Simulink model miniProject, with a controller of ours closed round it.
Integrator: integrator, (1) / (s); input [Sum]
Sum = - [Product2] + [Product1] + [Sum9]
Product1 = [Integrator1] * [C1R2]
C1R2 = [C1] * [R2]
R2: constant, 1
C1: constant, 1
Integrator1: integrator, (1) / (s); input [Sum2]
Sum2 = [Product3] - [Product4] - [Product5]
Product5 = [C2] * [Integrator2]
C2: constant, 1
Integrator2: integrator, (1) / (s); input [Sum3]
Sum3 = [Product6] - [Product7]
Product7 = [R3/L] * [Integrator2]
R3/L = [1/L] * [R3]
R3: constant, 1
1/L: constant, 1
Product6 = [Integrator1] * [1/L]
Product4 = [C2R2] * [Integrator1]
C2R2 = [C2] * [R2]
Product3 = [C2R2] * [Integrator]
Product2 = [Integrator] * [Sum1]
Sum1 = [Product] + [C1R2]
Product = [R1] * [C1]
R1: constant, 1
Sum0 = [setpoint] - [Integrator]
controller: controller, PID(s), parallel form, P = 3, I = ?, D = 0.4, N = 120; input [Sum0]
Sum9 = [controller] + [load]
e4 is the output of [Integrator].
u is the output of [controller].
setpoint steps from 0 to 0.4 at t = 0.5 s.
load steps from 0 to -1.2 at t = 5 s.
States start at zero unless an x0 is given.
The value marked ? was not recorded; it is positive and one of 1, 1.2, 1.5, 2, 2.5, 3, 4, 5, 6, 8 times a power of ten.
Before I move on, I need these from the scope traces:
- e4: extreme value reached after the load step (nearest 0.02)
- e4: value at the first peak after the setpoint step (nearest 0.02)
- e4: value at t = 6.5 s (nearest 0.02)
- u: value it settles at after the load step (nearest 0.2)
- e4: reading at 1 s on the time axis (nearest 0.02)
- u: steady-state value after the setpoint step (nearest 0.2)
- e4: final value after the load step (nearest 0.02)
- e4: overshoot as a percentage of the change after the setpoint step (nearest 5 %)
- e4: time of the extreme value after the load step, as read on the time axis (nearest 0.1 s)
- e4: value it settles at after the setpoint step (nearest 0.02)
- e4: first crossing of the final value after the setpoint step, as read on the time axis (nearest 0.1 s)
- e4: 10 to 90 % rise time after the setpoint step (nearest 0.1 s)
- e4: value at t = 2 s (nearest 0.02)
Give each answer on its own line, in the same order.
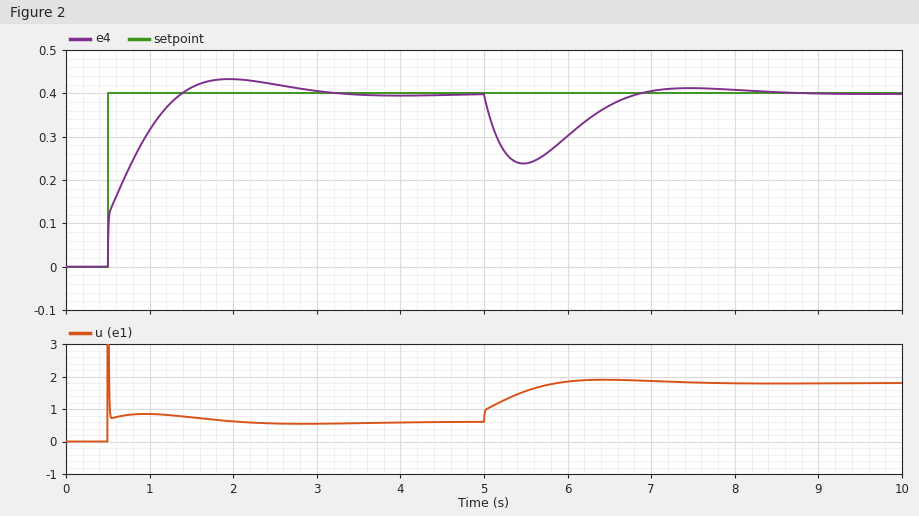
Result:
0.24
0.44
0.38
1.8
0.32
0.6
0.40
10 %
5.5 s
0.40
1.4 s
0.7 s
0.44
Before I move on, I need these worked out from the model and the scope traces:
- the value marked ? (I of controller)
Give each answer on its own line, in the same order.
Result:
8
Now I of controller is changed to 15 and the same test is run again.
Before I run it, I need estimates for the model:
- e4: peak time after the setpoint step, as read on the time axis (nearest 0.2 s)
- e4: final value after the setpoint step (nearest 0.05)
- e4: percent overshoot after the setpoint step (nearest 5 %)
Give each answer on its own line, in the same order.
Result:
1.4 s
0.40
15 %
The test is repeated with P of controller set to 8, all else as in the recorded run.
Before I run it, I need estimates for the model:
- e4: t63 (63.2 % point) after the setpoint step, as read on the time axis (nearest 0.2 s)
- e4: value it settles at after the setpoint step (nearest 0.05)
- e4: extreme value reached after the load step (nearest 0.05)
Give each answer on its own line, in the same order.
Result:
0.6 s
0.40
0.30
